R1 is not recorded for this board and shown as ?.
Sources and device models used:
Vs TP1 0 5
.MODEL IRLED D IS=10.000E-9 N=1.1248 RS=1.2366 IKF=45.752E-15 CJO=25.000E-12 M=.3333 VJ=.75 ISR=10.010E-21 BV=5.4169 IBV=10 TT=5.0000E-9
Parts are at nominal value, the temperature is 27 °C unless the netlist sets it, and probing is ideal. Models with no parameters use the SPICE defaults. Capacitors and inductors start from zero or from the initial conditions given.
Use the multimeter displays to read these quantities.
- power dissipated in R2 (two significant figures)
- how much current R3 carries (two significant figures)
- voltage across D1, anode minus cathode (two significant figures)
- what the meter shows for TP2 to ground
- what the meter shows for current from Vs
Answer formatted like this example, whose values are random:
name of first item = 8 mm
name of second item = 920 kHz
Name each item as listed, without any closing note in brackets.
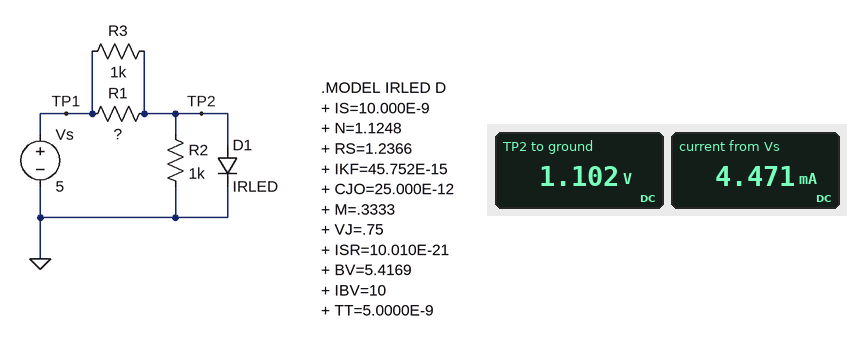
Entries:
power dissipated in R2 = 1.2 mW
how much current R3 carries = 3.9 mA
voltage across D1, anode minus cathode = 1.1 V
what the meter shows for TP2 to ground = 1.102 V
what the meter shows for current from Vs = 4.471 mA
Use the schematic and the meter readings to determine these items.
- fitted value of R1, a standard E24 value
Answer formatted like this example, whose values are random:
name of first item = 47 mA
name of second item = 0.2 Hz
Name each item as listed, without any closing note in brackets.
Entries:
fitted value of R1, a standard E24 value = 6.8 kΩ
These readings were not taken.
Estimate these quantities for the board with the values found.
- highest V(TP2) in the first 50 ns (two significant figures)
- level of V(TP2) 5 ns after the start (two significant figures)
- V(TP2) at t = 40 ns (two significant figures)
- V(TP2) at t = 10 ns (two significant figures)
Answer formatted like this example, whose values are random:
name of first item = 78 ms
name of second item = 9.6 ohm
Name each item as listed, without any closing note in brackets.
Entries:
highest V(TP2) in the first 50 ns = 1.1 V
level of V(TP2) 5 ns after the start = 750 mV
V(TP2) at t = 40 ns = 1.1 V
V(TP2) at t = 10 ns = 1.0 V
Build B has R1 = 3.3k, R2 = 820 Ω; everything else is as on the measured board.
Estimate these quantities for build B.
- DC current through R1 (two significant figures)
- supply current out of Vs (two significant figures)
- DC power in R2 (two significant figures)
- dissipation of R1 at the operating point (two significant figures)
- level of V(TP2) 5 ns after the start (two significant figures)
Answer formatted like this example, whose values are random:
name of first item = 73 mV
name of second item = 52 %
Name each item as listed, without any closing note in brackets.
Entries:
DC current through R1 = 1.2 mA
supply current out of Vs = 5.1 mA
DC power in R2 = 1.5 mW
dissipation of R1 at the operating point = 4.6 mW
level of V(TP2) 5 ns after the start = 810 mV
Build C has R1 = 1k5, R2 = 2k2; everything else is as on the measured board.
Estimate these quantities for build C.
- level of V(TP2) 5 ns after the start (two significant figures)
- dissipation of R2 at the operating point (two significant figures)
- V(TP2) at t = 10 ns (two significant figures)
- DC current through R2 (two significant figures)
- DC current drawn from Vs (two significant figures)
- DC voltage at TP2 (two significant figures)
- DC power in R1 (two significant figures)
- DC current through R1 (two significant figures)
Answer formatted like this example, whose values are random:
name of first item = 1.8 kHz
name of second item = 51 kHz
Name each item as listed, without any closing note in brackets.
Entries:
level of V(TP2) 5 ns after the start = 970 mV
dissipation of R2 at the operating point = 590 µW
V(TP2) at t = 10 ns = 1.1 V
DC current through R2 = 520 µA
DC current drawn from Vs = 6.4 mA
DC voltage at TP2 = 1.1 V
DC power in R1 = 9.9 mW
DC current through R1 = 2.6 mA
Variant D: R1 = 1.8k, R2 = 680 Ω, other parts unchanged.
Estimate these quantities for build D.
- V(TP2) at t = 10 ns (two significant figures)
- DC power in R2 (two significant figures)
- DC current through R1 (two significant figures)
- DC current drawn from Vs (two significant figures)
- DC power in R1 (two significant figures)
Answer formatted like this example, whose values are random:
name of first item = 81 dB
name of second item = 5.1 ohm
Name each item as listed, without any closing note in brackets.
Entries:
V(TP2) at t = 10 ns = 1.1 V
DC power in R2 = 1.8 mW
DC current through R1 = 2.2 mA
DC current drawn from Vs = 6.0 mA
DC power in R1 = 8.4 mW
